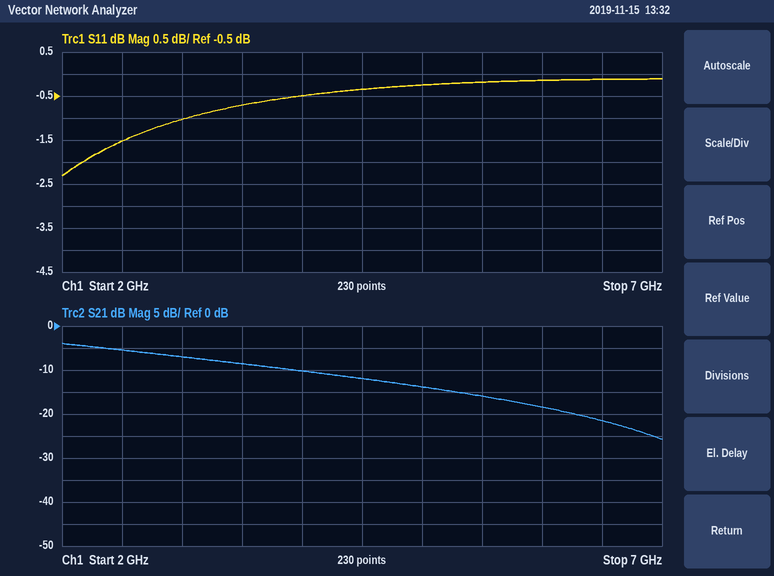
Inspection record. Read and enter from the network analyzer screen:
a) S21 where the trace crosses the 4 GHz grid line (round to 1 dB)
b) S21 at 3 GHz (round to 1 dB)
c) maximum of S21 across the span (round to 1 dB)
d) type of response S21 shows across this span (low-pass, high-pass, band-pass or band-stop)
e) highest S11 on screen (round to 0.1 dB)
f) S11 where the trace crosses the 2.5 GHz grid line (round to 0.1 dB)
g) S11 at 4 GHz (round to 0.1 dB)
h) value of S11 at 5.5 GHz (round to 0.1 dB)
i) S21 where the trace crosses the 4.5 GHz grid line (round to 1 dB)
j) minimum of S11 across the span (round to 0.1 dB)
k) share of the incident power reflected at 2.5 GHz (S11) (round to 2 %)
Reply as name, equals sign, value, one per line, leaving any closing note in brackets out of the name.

S21 where the trace crosses the 4 GHz grid line = -10 dB
S21 at 3 GHz = -7 dB
maximum of S21 across the span = -4 dB
type of response S21 shows across this span = low-pass
highest S11 on screen = -0.1 dB
S11 where the trace crosses the 2.5 GHz grid line = -1.5 dB
S11 at 4 GHz = -0.5 dB
value of S11 at 5.5 GHz = -0.2 dB
S21 where the trace crosses the 4.5 GHz grid line = -12 dB
minimum of S11 across the span = -2.3 dB
share of the incident power reflected at 2.5 GHz (S11) = 70 %
